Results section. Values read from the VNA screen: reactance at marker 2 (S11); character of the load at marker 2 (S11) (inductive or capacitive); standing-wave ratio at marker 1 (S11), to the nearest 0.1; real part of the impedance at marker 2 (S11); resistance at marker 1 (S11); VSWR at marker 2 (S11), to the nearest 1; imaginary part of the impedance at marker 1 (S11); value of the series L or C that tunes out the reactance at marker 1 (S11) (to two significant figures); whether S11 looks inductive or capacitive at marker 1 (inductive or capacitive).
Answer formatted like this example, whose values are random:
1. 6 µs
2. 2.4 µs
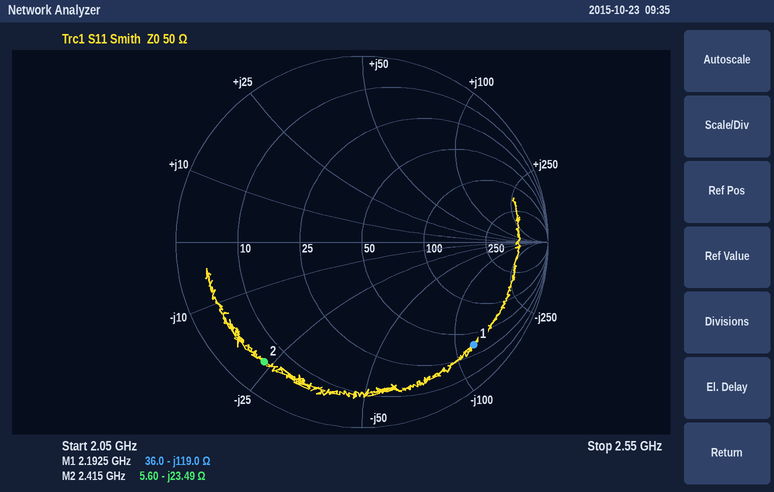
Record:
1. -23.49 Ω
2. capacitive
3. 9.9
4. 5.60 Ω
5. 36.0 Ω
6. 11
7. -119.0 Ω
8. 8.6 nH
9. capacitive
